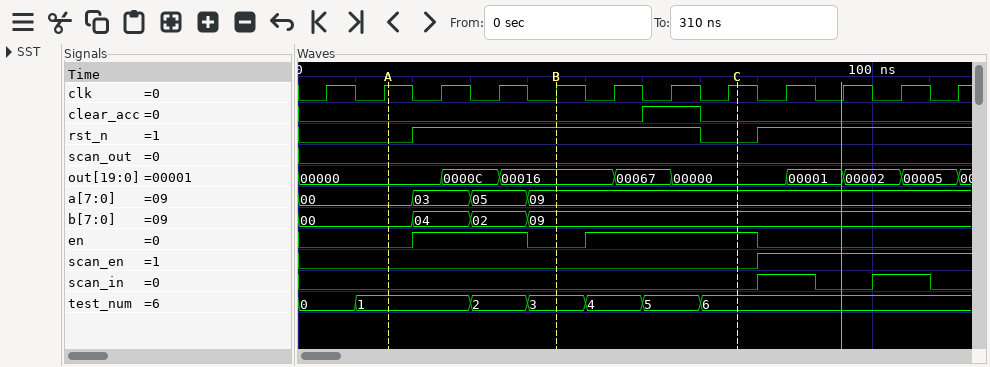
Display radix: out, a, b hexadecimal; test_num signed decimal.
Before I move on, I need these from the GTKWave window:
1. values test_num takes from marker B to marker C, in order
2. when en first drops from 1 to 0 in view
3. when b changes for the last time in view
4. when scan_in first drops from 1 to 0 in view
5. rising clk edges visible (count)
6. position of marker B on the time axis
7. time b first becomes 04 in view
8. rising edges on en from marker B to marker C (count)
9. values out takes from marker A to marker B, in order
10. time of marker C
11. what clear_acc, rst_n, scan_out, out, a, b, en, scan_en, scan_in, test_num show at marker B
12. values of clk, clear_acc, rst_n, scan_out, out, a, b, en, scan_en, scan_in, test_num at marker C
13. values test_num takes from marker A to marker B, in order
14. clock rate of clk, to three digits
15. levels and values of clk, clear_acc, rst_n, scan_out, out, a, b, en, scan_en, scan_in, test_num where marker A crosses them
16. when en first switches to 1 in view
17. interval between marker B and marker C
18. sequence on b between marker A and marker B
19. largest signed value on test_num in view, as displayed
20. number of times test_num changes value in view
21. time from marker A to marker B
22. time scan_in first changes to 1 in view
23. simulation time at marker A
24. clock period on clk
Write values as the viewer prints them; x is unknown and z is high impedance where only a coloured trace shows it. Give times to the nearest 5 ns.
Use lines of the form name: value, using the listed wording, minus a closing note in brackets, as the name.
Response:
values test_num takes from marker B to marker C, in order: 3, 4, 5, 6
when en first drops from 1 to 0 in view: 40 ns
when b changes for the last time in view: 40 ns
when scan_in first drops from 1 to 0 in view: 90 ns
rising clk edges visible: 12
position of marker B on the time axis: 45 ns
time b first becomes 04 in view: 20 ns
rising edges on en from marker B to marker C: 1
values out takes from marker A to marker B, in order: 00000, 0000C, 00016
time of marker C: 75 ns
what clear_acc, rst_n, scan_out, out, a, b, en, scan_en, scan_in, test_num show at marker B: clear_acc=0, rst_n=1, scan_out=0, out=00016, a=09, b=09, en=0, scan_en=0, scan_in=0, test_num=3
values of clk, clear_acc, rst_n, scan_out, out, a, b, en, scan_en, scan_in, test_num at marker C: clk=1, clear_acc=0, rst_n=0, scan_out=0, out=00000, a=09, b=09, en=1, scan_en=0, scan_in=0, test_num=6
values test_num takes from marker A to marker B, in order: 1, 2, 3
clock rate of clk, to three digits: 100 MHz
levels and values of clk, clear_acc, rst_n, scan_out, out, a, b, en, scan_en, scan_in, test_num where marker A crosses them: clk=1, clear_acc=0, rst_n=0, scan_out=0, out=00000, a=00, b=00, en=0, scan_en=0, scan_in=0, test_num=1
when en first switches to 1 in view: 20 ns
interval between marker B and marker C: 30 ns
sequence on b between marker A and marker B: 00, 04, 02, 09
largest signed value on test_num in view, as displayed: 6
number of times test_num changes value in view: 6
time from marker A to marker B: 30 ns
time scan_in first changes to 1 in view: 80 ns
simulation time at marker A: 15 ns
clock period on clk: 10 ns
